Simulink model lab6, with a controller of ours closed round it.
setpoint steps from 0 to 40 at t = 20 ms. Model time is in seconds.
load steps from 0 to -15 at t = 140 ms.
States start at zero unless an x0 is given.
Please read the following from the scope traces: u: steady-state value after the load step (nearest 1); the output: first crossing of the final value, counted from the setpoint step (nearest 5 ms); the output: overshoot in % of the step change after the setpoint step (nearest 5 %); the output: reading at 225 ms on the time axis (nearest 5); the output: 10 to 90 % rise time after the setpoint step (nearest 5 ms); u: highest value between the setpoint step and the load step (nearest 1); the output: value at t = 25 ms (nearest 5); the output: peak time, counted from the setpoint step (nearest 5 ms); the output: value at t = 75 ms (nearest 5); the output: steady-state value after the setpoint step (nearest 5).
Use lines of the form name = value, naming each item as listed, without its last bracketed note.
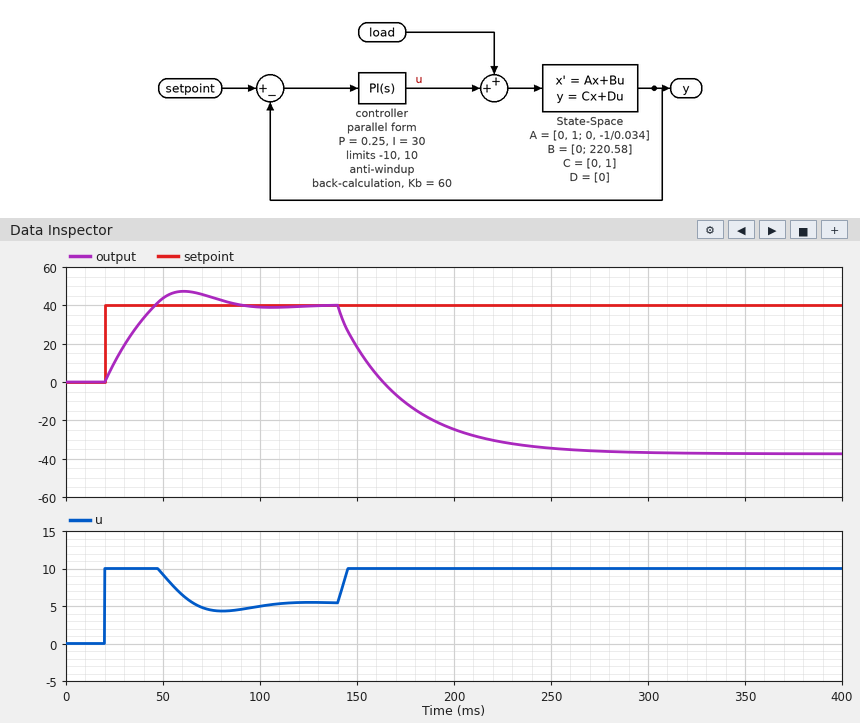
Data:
u: steady-state value after the load step = 10
the output: first crossing of the final value, counted from the setpoint step = 25 ms
the output: overshoot in % of the step change after the setpoint step = 20 %
the output: reading at 225 ms on the time axis = -30
the output: 10 to 90 % rise time after the setpoint step = 20 ms
u: highest value between the setpoint step and the load step = 10
the output: value at t = 25 ms = 10
the output: peak time, counted from the setpoint step = 40 ms
the output: value at t = 75 ms = 45
the output: steady-state value after the setpoint step = 40
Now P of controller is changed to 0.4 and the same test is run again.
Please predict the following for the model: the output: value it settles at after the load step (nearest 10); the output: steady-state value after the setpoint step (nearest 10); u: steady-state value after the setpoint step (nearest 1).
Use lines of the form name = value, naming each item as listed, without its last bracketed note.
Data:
the output: value it settles at after the load step = -40
the output: steady-state value after the setpoint step = 40
u: steady-state value after the setpoint step = 5
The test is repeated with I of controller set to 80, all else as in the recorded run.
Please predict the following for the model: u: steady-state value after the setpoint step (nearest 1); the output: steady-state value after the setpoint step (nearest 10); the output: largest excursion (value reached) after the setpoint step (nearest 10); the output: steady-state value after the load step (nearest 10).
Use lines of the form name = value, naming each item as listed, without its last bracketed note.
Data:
u: steady-state value after the setpoint step = 5
the output: steady-state value after the setpoint step = 40
the output: largest excursion (value reached) after the setpoint step = 50
the output: steady-state value after the load step = -40
